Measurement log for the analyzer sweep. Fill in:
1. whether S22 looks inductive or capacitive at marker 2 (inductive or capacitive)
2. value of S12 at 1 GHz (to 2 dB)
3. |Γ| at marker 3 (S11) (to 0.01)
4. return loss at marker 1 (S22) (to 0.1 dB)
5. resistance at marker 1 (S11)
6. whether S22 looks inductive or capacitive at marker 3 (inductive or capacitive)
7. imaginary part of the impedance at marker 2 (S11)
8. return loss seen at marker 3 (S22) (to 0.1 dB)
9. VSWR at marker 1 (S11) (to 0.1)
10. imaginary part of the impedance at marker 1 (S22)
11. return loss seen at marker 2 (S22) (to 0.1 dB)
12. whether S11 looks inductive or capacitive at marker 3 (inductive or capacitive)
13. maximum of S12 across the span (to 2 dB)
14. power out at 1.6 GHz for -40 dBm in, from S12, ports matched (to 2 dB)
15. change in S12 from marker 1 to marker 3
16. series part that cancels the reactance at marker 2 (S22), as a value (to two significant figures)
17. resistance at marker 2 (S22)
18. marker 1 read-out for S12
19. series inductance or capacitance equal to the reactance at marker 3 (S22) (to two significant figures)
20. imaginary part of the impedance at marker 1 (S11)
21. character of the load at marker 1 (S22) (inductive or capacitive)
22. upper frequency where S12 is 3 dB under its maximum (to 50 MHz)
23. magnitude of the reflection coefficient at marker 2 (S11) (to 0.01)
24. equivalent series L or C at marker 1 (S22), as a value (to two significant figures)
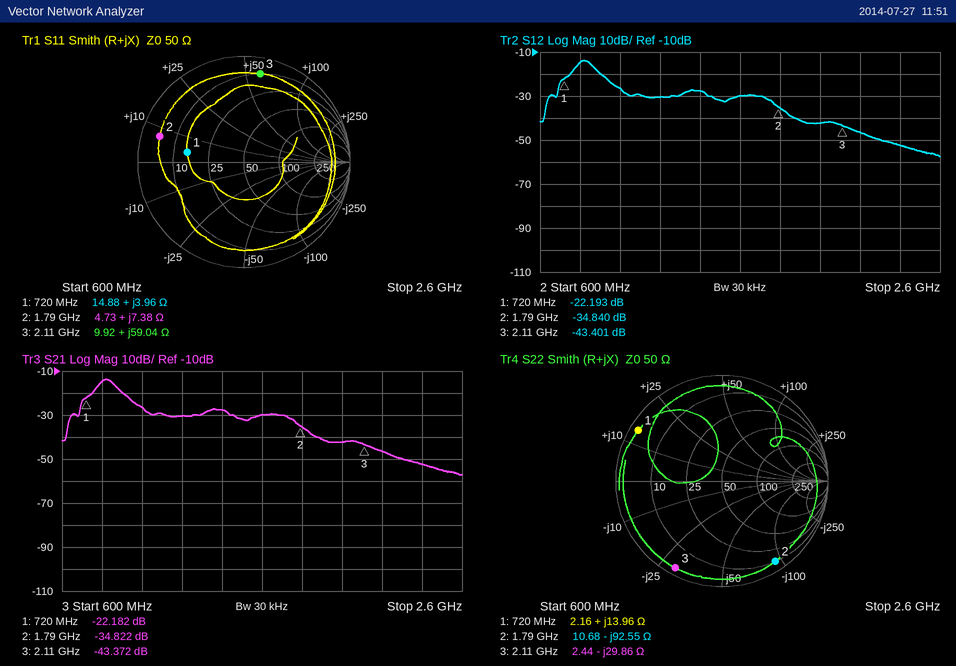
capacitive
-26 dB
0.85
0.7 dB
14.88 Ω
capacitive
+7.38 Ω
0.6 dB
3.4
+13.96 Ω
0.8 dB
inductive
-14 dB
-70 dBm
-21.208 dB
8.2 nH
10.68 Ω
-22.193 dB
2.5 pF
+3.96 Ω
inductive
850 MHz
0.83
3.1 nH
